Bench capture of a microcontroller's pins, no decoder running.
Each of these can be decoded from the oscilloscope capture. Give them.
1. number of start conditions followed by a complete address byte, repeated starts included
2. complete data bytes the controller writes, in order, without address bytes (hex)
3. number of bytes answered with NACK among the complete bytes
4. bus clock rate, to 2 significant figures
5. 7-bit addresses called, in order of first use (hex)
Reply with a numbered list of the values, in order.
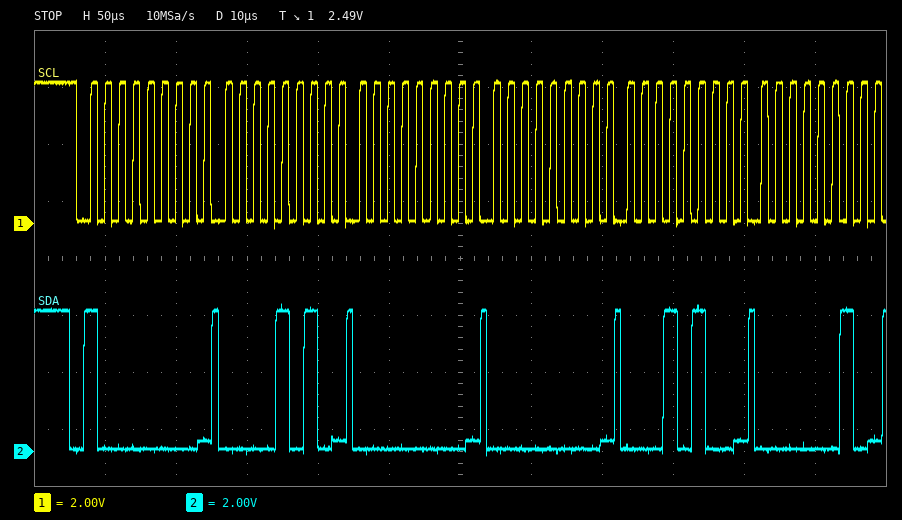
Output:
1. 1
2. 0A 00 00 14 02
3. 0
4. 100 kHz
5. 0x40
